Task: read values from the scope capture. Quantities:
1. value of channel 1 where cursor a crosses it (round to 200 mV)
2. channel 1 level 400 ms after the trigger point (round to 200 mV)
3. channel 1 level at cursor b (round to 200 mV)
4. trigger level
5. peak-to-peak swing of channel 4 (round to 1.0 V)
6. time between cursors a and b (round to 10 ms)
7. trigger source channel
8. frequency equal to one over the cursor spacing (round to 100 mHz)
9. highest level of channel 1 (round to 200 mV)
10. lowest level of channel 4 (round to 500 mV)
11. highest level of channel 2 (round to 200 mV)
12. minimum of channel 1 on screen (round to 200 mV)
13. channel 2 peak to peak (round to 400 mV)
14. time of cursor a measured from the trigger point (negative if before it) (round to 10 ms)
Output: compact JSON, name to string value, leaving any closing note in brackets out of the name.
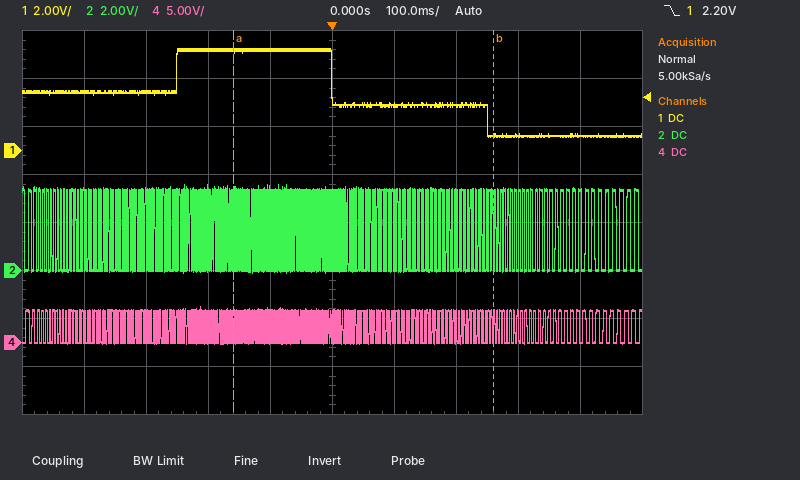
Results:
{"value of channel 1 where cursor a crosses it": "4.2 V", "channel 1 level 400 ms after the trigger point": "600 mV", "channel 1 level at cursor b": "600 mV", "trigger level": "2.20 V", "peak-to-peak swing of channel 4": "4.0 V", "time between cursors a and b": "420 ms", "trigger source channel": "channel 1", "frequency equal to one over the cursor spacing": "2.4 Hz", "highest level of channel 1": "4.2 V", "lowest level of channel 4": "0.0 V", "highest level of channel 2": "3.6 V", "minimum of channel 1 on screen": "600 mV", "channel 2 peak to peak": "3.6 V", "time of cursor a measured from the trigger point (negative if before it)": "-160 ms"}
